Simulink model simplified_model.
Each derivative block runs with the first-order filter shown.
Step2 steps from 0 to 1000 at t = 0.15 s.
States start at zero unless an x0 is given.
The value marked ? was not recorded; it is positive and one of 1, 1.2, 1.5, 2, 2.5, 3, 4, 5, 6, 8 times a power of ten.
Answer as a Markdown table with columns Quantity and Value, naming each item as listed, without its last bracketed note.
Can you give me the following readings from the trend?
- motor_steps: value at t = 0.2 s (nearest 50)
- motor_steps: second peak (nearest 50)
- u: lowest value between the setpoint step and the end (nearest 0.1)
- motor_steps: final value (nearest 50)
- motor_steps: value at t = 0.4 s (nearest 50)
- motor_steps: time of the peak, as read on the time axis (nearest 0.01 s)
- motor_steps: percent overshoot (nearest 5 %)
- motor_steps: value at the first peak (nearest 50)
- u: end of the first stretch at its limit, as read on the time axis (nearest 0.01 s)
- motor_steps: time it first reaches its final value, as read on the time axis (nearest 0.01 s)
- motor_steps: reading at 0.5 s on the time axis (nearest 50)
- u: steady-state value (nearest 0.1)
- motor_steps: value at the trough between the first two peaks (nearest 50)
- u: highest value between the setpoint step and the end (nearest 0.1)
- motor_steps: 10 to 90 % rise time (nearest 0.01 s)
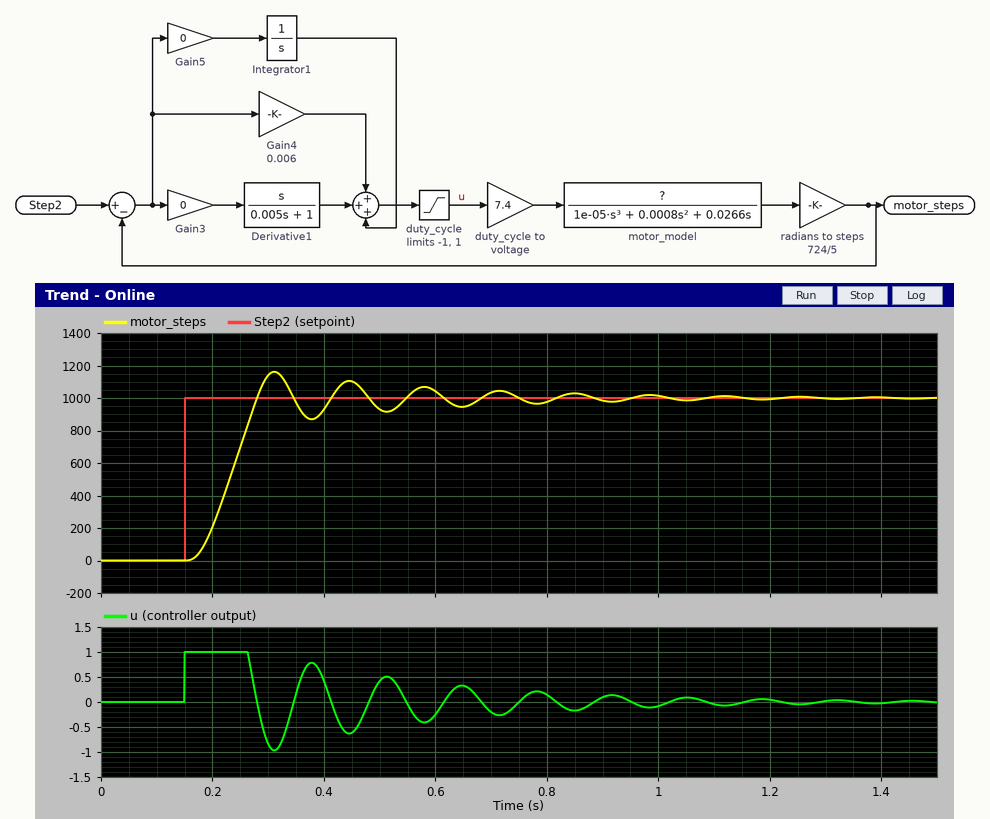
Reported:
| Quantity | Value |
|---|---|
| motor_steps: value at t = 0.2 s | 200 |
| motor_steps: second peak | 1100 |
| u: lowest value between the setpoint step and the end | -1.0 |
| motor_steps: final value | 1000 |
| motor_steps: value at t = 0.4 s | 950 |
| motor_steps: time of the peak, as read on the time axis | 0.31 s |
| motor_steps: percent overshoot | 15 % |
| motor_steps: value at the first peak | 1150 |
| u: end of the first stretch at its limit, as read on the time axis | 0.26 s |
| motor_steps: time it first reaches its final value, as read on the time axis | 0.28 s |
| motor_steps: reading at 0.5 s on the time axis | 950 |
| u: steady-state value | 0.0 |
| motor_steps: value at the trough between the first two peaks | 850 |
| u: highest value between the setpoint step and the end | 1.0 |
| motor_steps: 10 to 90 % rise time | 0.08 s |
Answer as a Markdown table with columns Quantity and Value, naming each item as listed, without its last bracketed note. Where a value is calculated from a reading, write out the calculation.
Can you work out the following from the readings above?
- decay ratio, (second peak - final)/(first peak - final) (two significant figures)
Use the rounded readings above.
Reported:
| Quantity | Value |
|---|---|
| decay ratio, (second peak - final)/(first peak - final) | (1100 - 1000) / (1150 - 1000) = 0.67 |
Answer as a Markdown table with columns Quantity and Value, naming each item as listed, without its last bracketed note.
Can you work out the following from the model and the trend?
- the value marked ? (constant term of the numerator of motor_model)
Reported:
| Quantity | Value |
|---|---|
| the value marked ? | 0.25 |
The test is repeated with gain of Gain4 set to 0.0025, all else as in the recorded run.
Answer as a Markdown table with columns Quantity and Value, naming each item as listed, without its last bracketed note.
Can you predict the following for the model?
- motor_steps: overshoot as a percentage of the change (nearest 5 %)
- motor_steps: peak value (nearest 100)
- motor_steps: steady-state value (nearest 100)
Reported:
| Quantity | Value |
|---|---|
| motor_steps: overshoot as a percentage of the change | 10 % |
| motor_steps: peak value | 1100 |
| motor_steps: steady-state value | 1000 |
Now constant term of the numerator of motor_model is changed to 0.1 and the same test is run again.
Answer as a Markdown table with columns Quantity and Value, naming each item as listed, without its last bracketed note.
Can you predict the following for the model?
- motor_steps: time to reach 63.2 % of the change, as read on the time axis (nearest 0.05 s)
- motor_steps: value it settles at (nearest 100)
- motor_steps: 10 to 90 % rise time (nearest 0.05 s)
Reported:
| Quantity | Value |
|---|---|
| motor_steps: time to reach 63.2 % of the change, as read on the time axis | 0.35 s |
| motor_steps: value it settles at | 1000 |
| motor_steps: 10 to 90 % rise time | 0.20 s |
